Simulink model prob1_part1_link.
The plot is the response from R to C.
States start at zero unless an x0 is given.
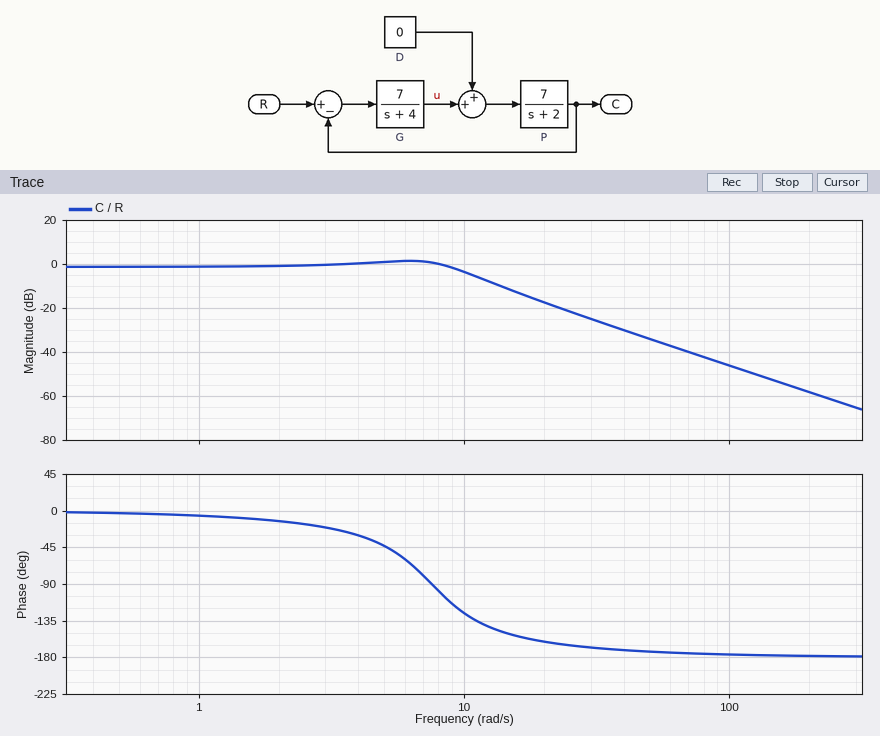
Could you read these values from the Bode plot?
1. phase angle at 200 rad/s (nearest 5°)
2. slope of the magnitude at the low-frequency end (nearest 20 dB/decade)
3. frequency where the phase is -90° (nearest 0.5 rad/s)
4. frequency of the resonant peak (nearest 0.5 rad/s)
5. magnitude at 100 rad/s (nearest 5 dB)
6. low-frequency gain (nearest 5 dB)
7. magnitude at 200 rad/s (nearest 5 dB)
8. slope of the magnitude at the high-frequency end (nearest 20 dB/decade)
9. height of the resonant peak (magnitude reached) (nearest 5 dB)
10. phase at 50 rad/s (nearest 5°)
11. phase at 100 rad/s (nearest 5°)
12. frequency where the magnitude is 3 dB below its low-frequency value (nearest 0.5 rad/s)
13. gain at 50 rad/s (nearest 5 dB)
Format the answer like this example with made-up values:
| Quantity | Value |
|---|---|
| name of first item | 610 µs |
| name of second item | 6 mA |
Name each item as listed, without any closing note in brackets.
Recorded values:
| Quantity | Value |
|---|---|
| phase angle at 200 rad/s | -180° |
| slope of the magnitude at the low-frequency end | 0 dB/decade |
| frequency where the phase is -90° | 7.5 rad/s |
| frequency of the resonant peak | 6.0 rad/s |
| magnitude at 100 rad/s | -45 dB |
| low-frequency gain | 0 dB |
| magnitude at 200 rad/s | -60 dB |
| slope of the magnitude at the high-frequency end | -40 dB/decade |
| height of the resonant peak (magnitude reached) | 0 dB |
| phase at 50 rad/s | -175° |
| phase at 100 rad/s | -175° |
| frequency where the magnitude is 3 dB below its low-frequency value | 10.5 rad/s |
| gain at 50 rad/s | -35 dB |
